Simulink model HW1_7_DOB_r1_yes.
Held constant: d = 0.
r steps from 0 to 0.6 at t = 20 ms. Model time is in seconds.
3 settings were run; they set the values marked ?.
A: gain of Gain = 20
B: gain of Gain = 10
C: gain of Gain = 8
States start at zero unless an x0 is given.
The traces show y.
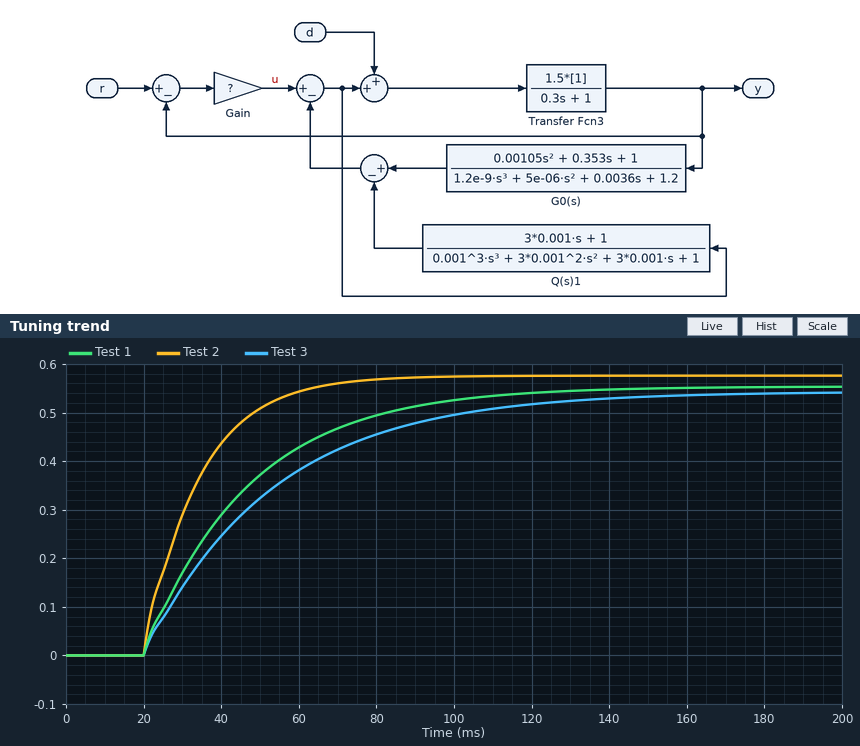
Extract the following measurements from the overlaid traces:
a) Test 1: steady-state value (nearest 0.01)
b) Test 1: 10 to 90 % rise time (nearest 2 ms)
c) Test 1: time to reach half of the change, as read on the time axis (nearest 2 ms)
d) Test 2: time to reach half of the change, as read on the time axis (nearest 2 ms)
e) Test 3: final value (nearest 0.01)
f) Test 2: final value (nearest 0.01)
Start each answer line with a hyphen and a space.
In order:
- 0.55
- 60 ms
- 38 ms
- 30 ms
- 0.54
- 0.58
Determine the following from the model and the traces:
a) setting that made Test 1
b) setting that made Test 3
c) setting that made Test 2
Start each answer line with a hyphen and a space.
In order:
- B
- C
- A
